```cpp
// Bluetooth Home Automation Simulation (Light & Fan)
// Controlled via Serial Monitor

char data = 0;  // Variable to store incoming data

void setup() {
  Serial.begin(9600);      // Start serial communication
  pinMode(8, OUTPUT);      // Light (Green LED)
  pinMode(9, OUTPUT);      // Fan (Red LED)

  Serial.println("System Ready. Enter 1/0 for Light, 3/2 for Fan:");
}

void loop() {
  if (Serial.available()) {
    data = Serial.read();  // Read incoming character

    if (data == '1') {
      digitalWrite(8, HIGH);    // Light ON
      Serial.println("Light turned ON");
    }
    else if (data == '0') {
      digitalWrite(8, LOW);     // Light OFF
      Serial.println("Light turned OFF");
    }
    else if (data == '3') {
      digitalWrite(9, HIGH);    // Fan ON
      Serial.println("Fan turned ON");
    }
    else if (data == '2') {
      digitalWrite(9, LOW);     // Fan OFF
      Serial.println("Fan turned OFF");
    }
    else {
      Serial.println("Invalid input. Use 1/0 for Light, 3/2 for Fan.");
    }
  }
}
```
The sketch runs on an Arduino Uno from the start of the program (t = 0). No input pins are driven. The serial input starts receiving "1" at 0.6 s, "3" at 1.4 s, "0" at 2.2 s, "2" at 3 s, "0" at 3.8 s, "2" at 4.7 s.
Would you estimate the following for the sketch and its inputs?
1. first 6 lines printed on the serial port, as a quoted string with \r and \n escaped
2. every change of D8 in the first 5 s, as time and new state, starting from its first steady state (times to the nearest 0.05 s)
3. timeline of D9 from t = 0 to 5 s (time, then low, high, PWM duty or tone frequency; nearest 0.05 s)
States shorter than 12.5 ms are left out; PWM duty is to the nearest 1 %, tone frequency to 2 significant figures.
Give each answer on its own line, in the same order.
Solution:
"System Ready. Enter 1/0 for Light, 3/2 for Fan:\r\nLight turned ON\r\nFan turned ON\r\nLight turned OFF\r\nFan turned OFF\r\nLight turned OFF\r\n"
0 s low; 0.6 s high; 2.2 s low
0 s low; 1.4 s high; 3 s low
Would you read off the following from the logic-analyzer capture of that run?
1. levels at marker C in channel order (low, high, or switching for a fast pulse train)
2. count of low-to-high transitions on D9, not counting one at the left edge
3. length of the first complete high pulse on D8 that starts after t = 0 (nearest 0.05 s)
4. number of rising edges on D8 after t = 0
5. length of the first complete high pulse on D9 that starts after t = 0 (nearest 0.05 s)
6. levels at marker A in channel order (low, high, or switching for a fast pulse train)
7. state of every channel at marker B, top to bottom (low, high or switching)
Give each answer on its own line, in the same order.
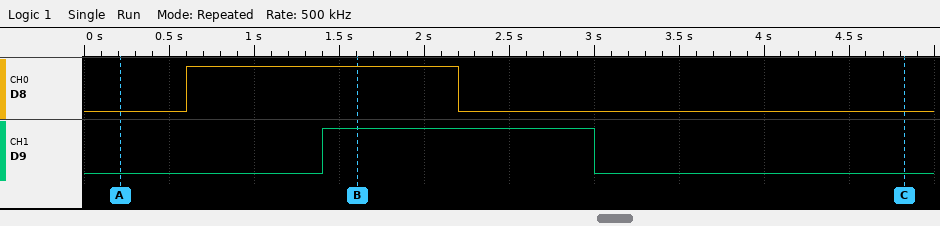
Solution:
D8 low, D9 low
1
1.60 s
1
1.60 s
D8 low, D9 low
D8 high, D9 high
